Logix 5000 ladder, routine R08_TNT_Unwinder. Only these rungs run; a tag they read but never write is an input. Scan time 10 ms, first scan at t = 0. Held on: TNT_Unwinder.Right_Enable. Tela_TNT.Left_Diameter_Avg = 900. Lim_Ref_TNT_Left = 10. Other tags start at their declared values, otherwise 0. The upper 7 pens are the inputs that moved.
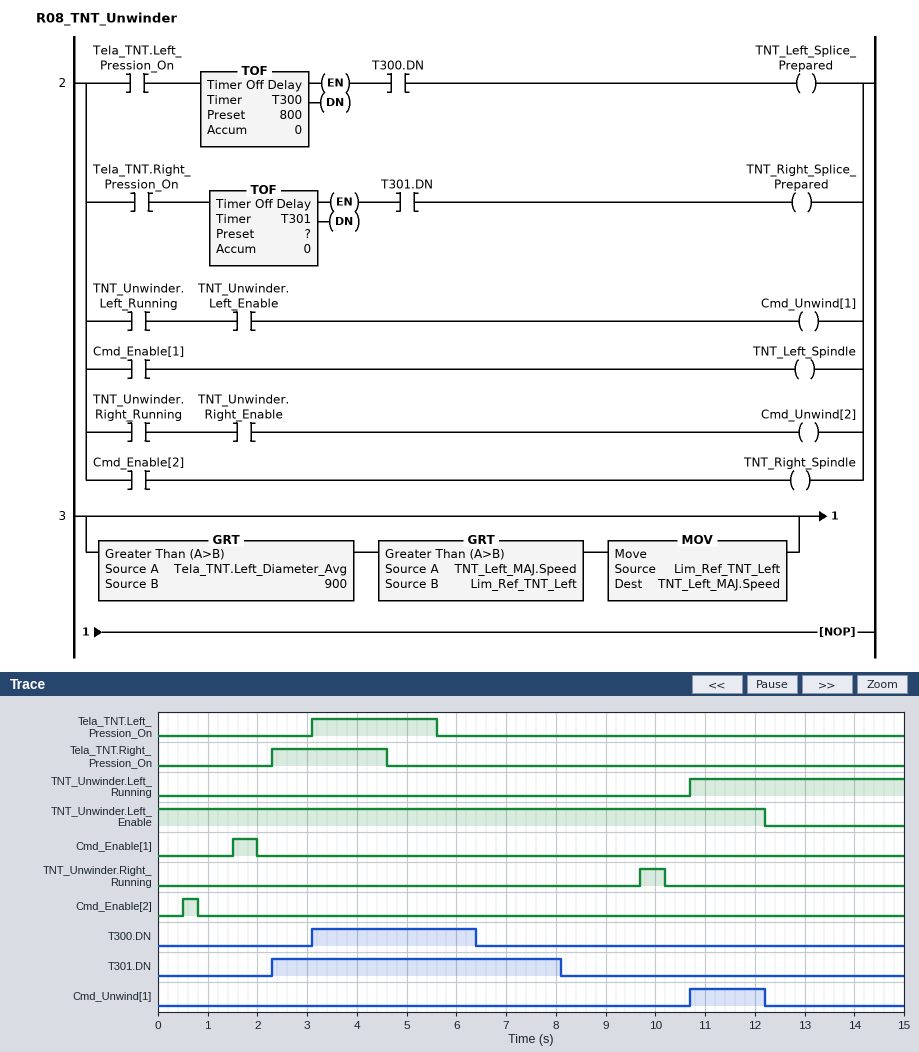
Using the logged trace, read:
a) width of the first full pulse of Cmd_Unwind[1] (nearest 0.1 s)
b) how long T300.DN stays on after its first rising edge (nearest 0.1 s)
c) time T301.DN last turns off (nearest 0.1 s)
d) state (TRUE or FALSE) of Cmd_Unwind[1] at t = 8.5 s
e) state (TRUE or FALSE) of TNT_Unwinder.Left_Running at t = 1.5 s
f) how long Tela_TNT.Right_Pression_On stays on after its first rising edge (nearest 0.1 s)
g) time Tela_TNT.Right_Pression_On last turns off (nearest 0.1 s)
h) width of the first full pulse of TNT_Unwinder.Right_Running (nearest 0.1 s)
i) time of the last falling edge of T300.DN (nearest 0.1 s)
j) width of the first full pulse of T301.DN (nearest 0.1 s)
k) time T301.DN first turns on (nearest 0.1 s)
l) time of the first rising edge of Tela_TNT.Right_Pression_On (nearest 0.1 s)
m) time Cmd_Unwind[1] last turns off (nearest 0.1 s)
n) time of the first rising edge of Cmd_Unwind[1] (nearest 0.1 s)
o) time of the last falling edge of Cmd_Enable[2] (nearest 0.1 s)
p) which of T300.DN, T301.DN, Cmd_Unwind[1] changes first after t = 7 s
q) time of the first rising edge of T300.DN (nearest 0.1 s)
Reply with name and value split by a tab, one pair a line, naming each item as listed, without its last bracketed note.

width of the first full pulse of Cmd_Unwind[1]	1.5 s
how long T300.DN stays on after its first rising edge	3.3 s
time T301.DN last turns off	8.1 s
state (TRUE or FALSE) of Cmd_Unwind[1] at t = 8.5 s	FALSE
state (TRUE or FALSE) of TNT_Unwinder.Left_Running at t = 1.5 s	FALSE
how long Tela_TNT.Right_Pression_On stays on after its first rising edge	2.3 s
time Tela_TNT.Right_Pression_On last turns off	4.6 s
width of the first full pulse of TNT_Unwinder.Right_Running	0.5 s
time of the last falling edge of T300.DN	6.4 s
width of the first full pulse of T301.DN	5.8 s
time T301.DN first turns on	2.3 s
time of the first rising edge of Tela_TNT.Right_Pression_On	2.3 s
time Cmd_Unwind[1] last turns off	12.2 s
time of the first rising edge of Cmd_Unwind[1]	10.7 s
time of the last falling edge of Cmd_Enable[2]	0.8 s
which of T300.DN, T301.DN, Cmd_Unwind[1] changes first after t = 7 s	T301.DN
time of the first rising edge of T300.DN	3.1 s
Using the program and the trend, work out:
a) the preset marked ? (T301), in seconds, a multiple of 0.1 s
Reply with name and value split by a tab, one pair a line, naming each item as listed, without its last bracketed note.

the preset marked ? (T301), in seconds, a multiple of 0.1 s	3.5 s
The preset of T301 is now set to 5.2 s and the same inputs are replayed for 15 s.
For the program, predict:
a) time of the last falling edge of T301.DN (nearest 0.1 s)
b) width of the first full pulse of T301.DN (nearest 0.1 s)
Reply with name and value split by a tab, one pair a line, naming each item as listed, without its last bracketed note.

time of the last falling edge of T301.DN	9.8 s
width of the first full pulse of T301.DN	7.5 s
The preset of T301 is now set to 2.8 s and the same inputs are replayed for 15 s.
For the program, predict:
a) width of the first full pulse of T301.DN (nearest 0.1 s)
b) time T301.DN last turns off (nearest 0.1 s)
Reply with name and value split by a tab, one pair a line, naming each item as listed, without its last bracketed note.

width of the first full pulse of T301.DN	5.1 s
time T301.DN last turns off	7.4 s
